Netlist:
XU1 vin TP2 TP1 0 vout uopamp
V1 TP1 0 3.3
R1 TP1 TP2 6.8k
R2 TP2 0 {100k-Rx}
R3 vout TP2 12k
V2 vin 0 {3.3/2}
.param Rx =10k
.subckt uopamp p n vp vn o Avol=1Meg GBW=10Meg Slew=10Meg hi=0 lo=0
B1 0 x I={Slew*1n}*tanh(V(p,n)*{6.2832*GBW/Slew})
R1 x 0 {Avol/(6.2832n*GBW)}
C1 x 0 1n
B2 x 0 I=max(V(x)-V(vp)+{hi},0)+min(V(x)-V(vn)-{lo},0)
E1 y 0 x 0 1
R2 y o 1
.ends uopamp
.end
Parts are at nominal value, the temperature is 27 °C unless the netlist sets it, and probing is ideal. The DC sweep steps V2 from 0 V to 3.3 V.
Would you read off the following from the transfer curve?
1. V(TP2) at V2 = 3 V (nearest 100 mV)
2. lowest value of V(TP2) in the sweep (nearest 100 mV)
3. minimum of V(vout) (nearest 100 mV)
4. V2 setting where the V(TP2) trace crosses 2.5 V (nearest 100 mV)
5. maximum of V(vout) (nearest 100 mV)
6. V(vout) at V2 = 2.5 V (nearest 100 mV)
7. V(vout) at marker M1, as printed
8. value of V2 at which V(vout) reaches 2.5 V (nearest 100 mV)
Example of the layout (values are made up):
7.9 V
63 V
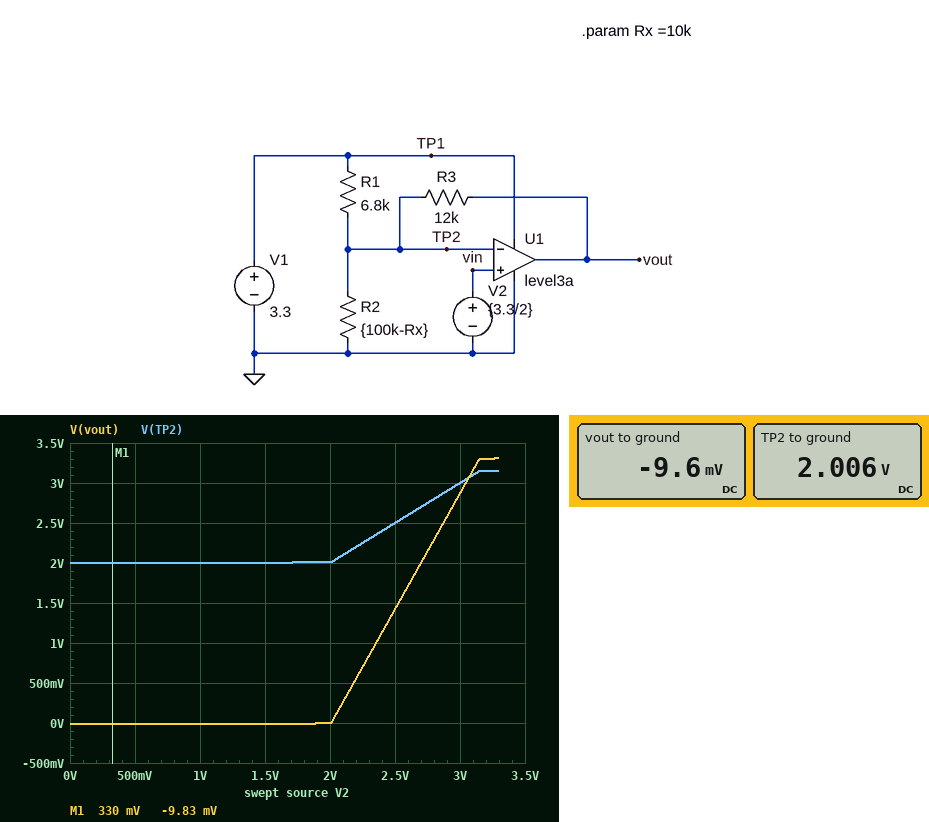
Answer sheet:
3.0 V
2.0 V
0 V
2.5 V
3.3 V
1.4 V
-9.83 mV
2.9 V
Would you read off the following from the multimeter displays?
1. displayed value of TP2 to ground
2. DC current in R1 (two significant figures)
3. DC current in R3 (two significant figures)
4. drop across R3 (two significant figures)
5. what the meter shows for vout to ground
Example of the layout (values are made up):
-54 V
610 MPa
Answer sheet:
2.006 V
190 µA
170 µA
2.0 V
-9.6 mV
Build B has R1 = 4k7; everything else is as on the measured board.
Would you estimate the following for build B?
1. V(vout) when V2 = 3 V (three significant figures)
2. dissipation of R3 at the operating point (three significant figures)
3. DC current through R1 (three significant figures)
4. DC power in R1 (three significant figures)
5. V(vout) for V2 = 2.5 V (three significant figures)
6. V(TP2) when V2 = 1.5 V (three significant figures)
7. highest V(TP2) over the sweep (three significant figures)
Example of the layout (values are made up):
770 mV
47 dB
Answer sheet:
2.63 V
438 µW
216 µA
220 µW
791 mV
2.28 V
3.18 V
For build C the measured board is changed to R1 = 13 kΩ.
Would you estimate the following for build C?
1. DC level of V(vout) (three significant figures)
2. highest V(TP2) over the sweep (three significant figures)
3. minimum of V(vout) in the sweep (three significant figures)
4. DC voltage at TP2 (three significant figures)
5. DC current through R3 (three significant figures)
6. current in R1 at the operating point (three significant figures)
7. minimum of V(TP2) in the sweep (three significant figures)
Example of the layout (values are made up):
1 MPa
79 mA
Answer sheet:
347 mV
3.09 V
-9.88 mV
1.65 V
109 µA
127 µA
1.48 V
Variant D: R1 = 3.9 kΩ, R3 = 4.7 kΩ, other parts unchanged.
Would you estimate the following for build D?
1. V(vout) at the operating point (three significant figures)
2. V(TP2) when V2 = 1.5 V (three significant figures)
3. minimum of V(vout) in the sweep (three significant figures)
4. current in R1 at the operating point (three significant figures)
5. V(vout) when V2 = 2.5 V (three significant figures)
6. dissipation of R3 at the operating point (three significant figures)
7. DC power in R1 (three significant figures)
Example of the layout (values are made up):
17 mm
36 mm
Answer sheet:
-5.58 mV
1.76 V
-9.62 mV
395 µA
1.67 V
663 µW
609 µW
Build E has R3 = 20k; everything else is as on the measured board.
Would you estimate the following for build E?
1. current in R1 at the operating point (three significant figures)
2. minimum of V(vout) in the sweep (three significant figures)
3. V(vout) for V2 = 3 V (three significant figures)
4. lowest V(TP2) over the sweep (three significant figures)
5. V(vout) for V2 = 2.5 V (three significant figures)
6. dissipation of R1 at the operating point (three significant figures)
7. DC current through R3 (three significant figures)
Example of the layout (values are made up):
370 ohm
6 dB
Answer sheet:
143 µA
-9.88 mV
2.78 V
2.33 V
703 mV
139 µW
117 µA
